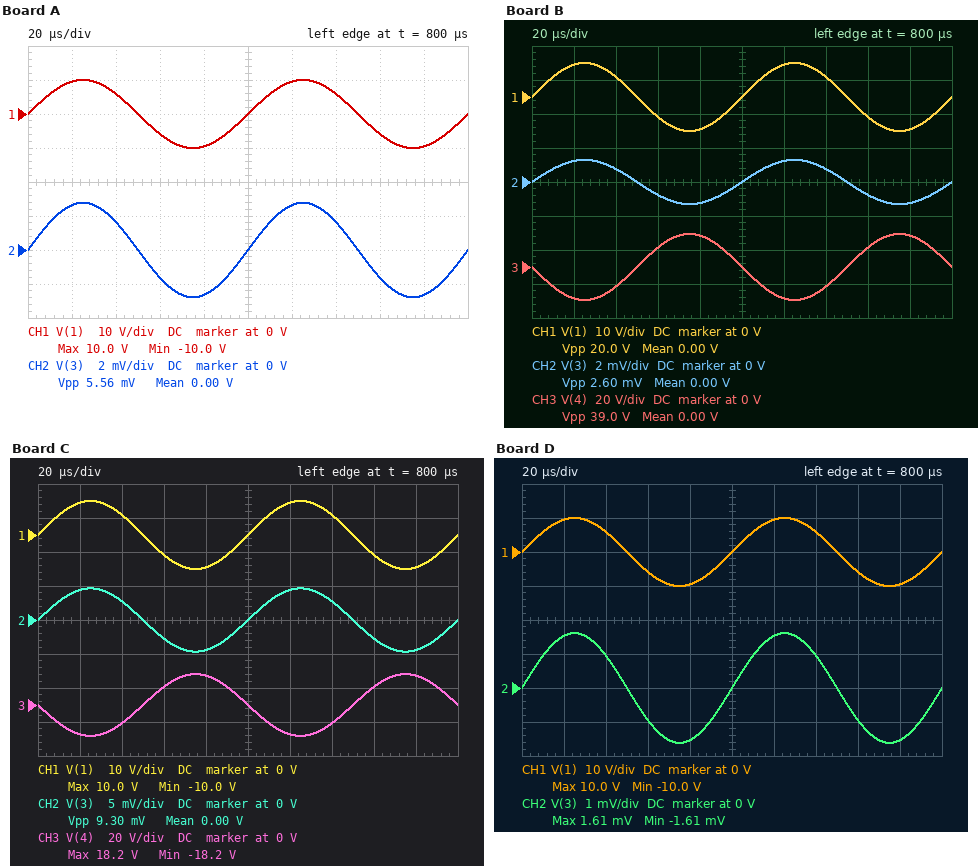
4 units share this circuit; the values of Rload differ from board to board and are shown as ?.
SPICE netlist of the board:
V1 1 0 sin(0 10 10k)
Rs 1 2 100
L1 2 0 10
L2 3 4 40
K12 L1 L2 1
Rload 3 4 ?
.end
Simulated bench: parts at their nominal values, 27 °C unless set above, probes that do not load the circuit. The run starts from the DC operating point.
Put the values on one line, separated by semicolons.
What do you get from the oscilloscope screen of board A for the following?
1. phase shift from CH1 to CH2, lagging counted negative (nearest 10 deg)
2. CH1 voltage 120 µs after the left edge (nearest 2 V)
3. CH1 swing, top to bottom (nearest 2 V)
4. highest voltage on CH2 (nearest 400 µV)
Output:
0 deg; 10 V; 20 V; 2.8 mV
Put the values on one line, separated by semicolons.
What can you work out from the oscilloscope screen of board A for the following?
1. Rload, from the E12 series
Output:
6.8 kΩ
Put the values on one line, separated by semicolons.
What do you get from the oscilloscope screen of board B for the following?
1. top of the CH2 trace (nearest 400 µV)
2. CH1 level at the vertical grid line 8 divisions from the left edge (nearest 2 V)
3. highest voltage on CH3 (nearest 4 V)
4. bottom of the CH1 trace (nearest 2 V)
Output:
1.2 mV; -6 V; 20 V; -10 V
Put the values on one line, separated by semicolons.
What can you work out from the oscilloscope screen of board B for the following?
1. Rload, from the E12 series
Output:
15 kΩ
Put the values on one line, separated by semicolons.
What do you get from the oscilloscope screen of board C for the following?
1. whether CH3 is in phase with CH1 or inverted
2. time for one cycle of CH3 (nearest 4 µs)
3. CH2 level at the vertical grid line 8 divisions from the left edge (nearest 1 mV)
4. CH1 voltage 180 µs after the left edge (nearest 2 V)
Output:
inverted; 100 µs; -3 mV; -10 V
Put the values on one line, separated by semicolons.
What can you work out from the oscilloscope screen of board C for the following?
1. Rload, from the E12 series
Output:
3.9 kΩ
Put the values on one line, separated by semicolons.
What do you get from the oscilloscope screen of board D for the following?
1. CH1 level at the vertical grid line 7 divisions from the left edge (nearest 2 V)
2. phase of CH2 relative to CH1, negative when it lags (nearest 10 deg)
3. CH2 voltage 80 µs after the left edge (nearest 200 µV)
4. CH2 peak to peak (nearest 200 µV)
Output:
6 V; 0 deg; -1.6 mV; 3.2 mV
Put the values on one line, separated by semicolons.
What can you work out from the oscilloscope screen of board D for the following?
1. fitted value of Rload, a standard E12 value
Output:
12 kΩ
